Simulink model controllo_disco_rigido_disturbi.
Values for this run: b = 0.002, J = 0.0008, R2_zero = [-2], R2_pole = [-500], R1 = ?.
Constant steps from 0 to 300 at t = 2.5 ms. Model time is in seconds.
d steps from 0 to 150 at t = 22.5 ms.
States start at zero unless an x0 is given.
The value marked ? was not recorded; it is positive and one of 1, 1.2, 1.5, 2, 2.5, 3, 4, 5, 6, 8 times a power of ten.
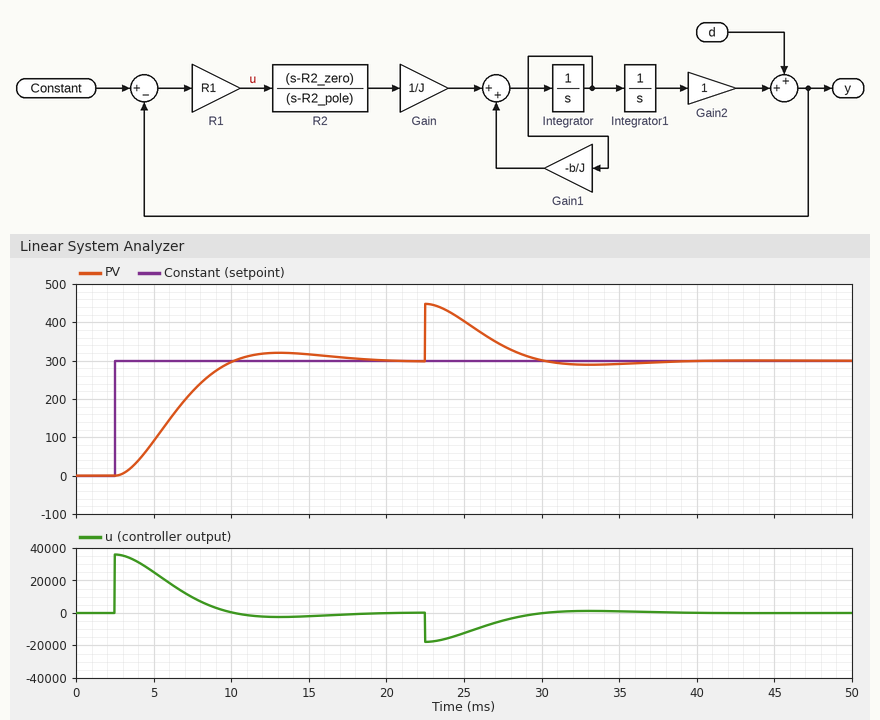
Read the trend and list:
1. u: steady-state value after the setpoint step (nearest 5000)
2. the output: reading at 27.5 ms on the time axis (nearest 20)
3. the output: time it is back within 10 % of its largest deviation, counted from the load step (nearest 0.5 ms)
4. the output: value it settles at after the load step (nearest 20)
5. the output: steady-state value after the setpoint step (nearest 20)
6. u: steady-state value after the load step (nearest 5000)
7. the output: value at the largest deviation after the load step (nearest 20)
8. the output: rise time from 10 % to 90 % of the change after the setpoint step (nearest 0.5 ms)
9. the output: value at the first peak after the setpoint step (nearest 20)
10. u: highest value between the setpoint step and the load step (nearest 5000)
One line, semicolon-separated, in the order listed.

0; 340; 6.5 ms; 300; 300; 0; 440; 5.0 ms; 320; 35000
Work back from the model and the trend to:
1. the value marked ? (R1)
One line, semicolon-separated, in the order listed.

120
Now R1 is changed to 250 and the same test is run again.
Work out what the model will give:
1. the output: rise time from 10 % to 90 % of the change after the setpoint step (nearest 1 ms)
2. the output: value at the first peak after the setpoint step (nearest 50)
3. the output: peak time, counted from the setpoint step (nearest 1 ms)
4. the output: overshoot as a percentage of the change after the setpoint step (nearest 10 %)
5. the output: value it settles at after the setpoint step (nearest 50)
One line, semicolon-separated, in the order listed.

3 ms; 350; 6 ms; 20 %; 300
